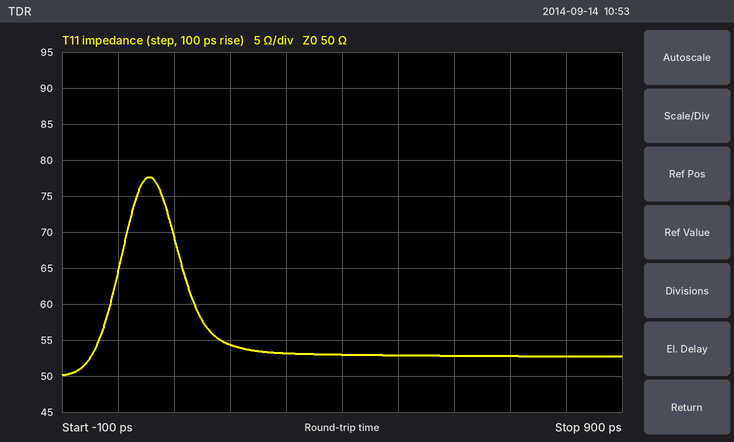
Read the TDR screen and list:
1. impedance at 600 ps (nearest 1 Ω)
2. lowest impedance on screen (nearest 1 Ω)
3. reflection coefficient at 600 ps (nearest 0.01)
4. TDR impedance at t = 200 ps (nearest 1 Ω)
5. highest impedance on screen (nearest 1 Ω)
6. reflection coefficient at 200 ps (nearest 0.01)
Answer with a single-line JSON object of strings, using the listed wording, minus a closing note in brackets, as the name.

{"impedance at 600 ps": "53 Ω", "lowest impedance on screen": "50 Ω", "reflection coefficient at 600 ps": "+0.03", "TDR impedance at t = 200 ps": "54 Ω", "highest impedance on screen": "78 Ω", "reflection coefficient at 200 ps": "+0.04"}
